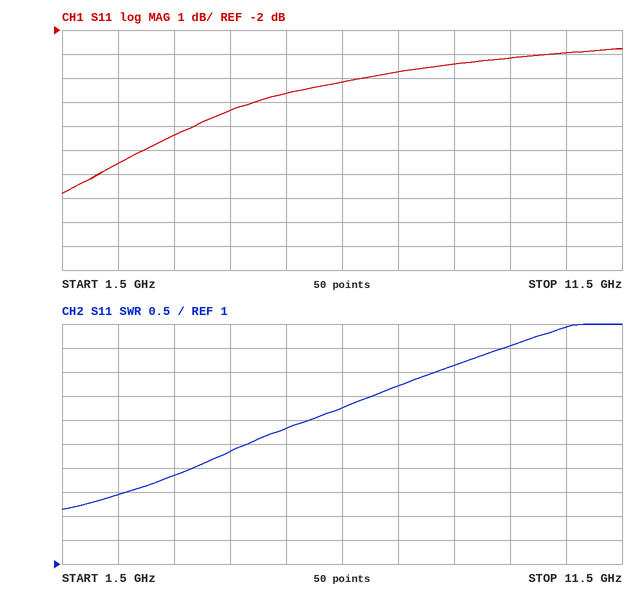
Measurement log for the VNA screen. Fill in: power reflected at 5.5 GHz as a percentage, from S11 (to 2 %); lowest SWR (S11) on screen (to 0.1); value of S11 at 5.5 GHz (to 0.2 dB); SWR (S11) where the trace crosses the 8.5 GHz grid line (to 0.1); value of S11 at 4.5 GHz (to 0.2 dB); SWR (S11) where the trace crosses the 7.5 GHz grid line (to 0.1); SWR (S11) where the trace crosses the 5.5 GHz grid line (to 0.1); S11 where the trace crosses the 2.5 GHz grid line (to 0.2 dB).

34 %
2.1
-4.6 dB
5.1
-5.4 dB
4.7
3.8
-7.6 dB
